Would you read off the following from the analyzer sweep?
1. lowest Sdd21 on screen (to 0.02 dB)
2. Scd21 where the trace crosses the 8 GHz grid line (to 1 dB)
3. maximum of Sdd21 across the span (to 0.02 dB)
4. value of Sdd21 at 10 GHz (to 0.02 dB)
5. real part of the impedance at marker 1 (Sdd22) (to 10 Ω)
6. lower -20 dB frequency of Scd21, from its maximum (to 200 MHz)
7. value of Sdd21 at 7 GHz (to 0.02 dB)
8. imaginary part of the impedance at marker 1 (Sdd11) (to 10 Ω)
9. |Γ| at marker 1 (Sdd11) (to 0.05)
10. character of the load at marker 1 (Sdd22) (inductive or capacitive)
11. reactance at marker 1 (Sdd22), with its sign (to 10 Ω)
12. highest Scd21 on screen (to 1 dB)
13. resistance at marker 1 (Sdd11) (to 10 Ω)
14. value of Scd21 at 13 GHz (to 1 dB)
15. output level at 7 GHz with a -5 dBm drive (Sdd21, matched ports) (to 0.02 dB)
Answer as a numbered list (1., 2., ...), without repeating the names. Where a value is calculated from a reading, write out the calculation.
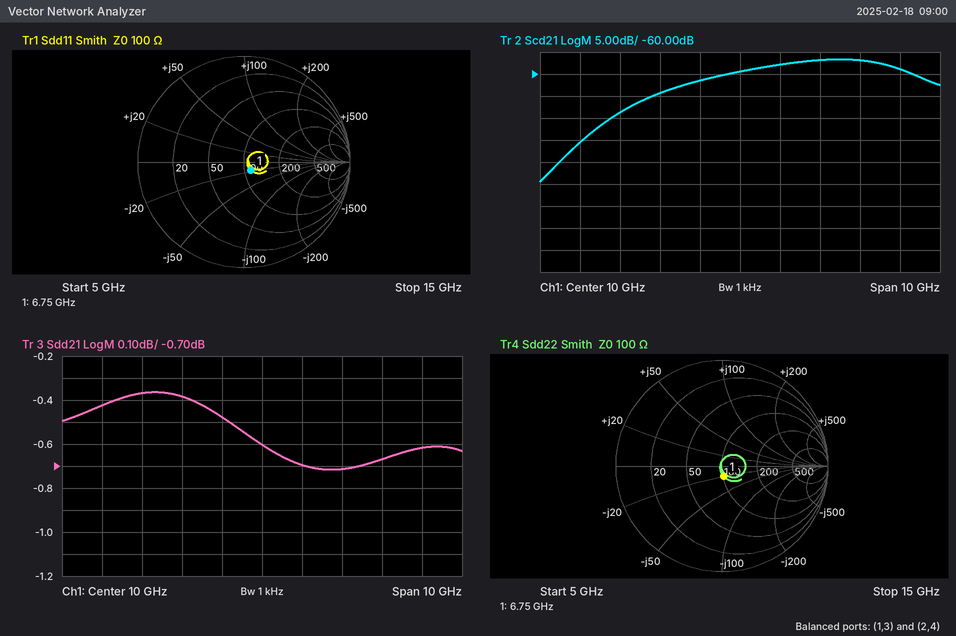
1. -0.72 dB
2. -64 dB
3. -0.36 dB
4. -0.60 dB
5. 100 Ω
6. 5.8 GHz
7. -0.36 dB
8. -20 Ω
9. 0.10
10. capacitive
11. -20 Ω
12. -57 dB
13. 110 Ω
14. -57 dB
15. -5 dBm + (-0.36 dB) = -5.36 dBm
